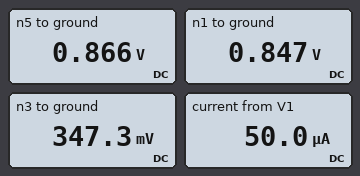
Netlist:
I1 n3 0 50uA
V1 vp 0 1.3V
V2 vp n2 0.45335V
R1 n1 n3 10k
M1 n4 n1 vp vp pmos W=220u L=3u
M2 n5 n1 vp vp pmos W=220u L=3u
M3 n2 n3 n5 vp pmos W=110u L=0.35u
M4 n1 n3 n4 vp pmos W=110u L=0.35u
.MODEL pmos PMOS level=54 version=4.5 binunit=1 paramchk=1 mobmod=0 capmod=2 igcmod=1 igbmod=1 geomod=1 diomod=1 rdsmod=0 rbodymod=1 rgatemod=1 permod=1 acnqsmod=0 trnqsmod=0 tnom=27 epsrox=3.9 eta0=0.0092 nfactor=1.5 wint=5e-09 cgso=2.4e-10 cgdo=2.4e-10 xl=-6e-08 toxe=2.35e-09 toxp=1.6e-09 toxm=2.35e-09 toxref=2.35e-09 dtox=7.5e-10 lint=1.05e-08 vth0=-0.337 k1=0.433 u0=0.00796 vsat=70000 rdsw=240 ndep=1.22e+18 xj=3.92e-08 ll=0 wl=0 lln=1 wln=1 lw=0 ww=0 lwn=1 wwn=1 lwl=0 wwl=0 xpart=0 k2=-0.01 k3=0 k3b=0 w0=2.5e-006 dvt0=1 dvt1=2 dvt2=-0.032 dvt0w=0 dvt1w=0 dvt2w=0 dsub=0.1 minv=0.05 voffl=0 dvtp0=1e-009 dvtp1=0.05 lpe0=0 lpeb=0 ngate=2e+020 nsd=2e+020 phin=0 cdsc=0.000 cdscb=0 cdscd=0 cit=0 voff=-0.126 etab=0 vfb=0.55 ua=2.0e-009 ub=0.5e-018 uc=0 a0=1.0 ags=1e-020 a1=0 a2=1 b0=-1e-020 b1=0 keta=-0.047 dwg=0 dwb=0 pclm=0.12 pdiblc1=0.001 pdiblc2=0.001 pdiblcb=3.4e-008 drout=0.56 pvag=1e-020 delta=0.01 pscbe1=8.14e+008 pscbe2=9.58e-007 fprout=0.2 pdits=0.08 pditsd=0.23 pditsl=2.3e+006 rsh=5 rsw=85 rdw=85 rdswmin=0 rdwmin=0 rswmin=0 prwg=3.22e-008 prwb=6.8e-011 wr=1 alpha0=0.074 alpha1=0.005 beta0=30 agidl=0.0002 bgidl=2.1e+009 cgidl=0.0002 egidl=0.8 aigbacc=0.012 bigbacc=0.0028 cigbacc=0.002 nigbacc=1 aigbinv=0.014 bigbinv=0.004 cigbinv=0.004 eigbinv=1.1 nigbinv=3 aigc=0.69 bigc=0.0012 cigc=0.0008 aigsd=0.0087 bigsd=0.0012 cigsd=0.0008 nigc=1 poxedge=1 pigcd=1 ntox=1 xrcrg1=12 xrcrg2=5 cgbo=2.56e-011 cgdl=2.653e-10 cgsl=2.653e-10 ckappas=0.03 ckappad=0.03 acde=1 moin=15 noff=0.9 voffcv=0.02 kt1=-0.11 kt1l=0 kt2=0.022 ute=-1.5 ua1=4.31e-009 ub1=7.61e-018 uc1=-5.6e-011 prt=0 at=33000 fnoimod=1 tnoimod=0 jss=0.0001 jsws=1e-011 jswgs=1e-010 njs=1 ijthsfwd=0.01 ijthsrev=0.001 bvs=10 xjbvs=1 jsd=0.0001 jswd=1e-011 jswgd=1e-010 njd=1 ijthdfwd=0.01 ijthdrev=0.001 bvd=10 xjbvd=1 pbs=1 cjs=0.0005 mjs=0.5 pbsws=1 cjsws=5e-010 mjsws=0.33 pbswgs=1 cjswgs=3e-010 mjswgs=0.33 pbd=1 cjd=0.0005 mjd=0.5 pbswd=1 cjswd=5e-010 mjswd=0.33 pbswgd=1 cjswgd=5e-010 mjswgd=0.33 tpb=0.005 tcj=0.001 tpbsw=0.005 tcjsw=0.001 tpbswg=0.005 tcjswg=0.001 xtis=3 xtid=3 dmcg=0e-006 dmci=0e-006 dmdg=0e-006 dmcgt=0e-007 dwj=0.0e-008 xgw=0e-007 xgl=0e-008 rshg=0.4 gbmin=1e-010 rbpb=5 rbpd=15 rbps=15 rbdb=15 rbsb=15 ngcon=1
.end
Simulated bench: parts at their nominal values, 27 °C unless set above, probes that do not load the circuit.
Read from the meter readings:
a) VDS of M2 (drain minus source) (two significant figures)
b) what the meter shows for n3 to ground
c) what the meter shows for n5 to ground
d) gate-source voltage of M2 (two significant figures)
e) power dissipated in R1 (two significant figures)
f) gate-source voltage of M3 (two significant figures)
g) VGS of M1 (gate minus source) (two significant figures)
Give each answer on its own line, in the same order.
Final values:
-430 mV
347.3 mV
0.866 V
-450 mV
25 µW
-520 mV
-450 mV
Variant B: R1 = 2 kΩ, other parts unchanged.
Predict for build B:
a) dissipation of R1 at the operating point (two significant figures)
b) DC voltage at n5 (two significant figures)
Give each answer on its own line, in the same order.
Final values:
5.0 µW
1.1 V
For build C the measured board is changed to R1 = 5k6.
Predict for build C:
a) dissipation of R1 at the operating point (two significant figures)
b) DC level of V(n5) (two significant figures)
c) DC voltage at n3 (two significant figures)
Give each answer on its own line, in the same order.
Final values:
14 µW
980 mV
570 mV
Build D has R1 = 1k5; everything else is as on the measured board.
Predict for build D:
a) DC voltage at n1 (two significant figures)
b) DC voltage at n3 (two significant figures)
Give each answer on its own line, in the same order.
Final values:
840 mV
770 mV
